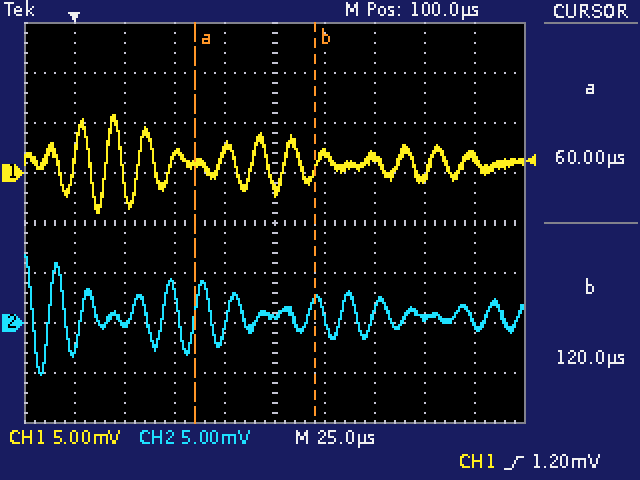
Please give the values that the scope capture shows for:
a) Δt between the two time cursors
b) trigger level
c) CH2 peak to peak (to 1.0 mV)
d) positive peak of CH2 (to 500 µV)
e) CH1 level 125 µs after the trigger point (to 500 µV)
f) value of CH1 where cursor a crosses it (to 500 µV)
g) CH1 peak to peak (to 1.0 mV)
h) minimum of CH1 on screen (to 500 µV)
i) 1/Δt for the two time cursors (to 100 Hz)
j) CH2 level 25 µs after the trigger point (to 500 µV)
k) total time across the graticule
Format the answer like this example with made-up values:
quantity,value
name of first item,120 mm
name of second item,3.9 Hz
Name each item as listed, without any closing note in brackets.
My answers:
quantity,value
Δt between the two time cursors,60.0 µs
trigger level,1.20 mV
CH2 peak to peak,12.0 mV
positive peak of CH2,7.0 mV
CH1 level 125 µs after the trigger point,2.0 mV
value of CH1 where cursor a crosses it,1.0 mV
CH1 peak to peak,10.0 mV
minimum of CH1 on screen,-4.0 mV
1/Δt for the two time cursors,16.7 kHz
CH2 level 25 µs after the trigger point,0.0 mV
total time across the graticule,250 µs
